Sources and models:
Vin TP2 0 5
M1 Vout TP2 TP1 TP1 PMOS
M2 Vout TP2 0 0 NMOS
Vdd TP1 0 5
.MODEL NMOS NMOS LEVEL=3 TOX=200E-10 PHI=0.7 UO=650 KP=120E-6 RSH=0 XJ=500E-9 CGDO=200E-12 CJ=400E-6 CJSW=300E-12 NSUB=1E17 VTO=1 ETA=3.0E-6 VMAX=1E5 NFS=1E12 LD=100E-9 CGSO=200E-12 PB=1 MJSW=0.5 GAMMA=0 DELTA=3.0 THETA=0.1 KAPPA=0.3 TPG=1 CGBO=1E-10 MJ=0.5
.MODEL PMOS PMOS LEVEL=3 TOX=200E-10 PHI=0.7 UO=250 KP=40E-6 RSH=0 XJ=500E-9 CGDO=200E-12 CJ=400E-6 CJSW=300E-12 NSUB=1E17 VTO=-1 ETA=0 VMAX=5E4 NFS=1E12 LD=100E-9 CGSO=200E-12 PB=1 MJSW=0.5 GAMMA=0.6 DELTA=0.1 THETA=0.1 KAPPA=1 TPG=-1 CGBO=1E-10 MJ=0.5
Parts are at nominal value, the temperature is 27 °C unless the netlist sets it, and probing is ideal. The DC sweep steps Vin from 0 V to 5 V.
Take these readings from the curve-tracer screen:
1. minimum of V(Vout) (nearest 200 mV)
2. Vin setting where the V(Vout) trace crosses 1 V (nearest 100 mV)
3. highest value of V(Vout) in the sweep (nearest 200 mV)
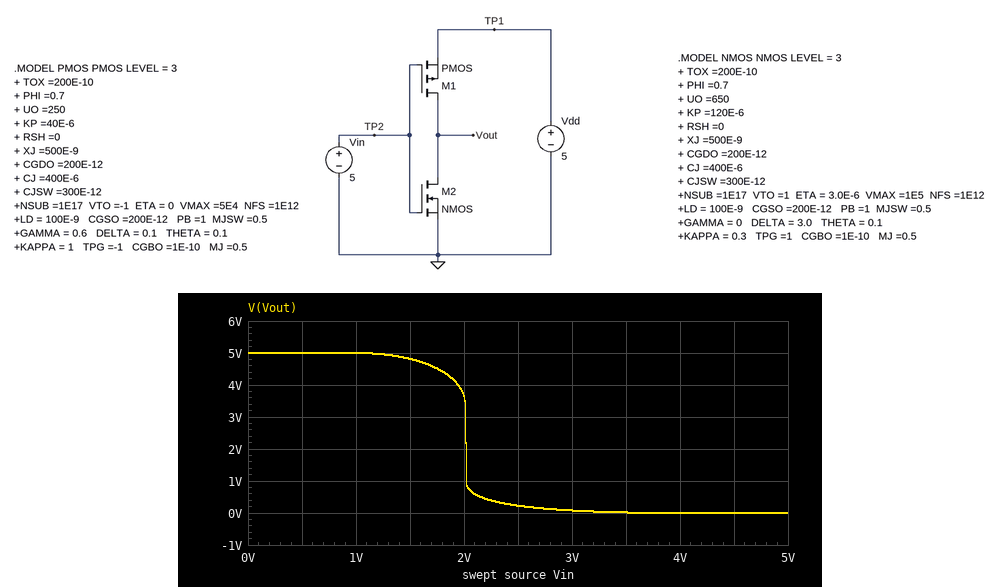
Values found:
0 V
2.0 V
5.0 V
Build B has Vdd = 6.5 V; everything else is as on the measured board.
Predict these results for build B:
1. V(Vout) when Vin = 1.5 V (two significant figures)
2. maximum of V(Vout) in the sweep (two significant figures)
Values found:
6.4 V
6.5 V
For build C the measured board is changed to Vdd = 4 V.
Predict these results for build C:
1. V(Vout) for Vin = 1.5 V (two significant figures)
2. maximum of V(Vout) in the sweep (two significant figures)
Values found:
3.7 V
4.0 V
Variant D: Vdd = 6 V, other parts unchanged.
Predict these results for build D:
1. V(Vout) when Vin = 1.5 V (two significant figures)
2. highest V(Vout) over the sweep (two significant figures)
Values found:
5.9 V
6.0 V
